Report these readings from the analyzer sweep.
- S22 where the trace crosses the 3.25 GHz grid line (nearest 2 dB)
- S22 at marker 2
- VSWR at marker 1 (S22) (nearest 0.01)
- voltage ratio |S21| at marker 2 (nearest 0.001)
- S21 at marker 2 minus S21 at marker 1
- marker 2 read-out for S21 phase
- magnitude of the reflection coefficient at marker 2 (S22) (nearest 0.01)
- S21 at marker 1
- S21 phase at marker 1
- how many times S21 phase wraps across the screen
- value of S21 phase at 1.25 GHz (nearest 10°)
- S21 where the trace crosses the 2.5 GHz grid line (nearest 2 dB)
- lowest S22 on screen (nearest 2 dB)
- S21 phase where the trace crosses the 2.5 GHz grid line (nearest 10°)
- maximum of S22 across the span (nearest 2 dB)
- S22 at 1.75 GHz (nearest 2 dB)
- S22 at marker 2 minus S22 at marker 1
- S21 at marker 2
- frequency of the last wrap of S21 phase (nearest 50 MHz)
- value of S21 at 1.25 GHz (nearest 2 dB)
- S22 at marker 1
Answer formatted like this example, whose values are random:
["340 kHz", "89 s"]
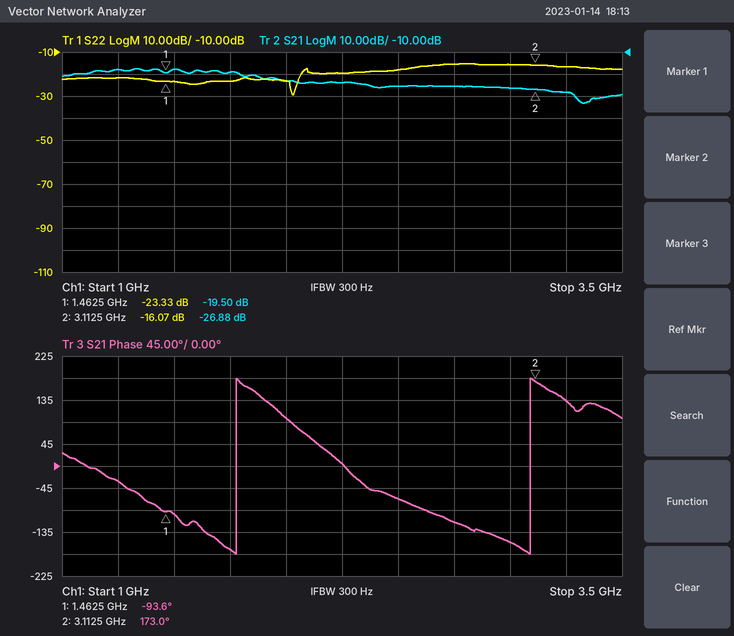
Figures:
["-16 dB", "-16.07 dB", "1.15", "0.045", "-7.38 dB", "173.0°", "0.16", "-19.50 dB", "-93.6°", "2", "-30°", "-26 dB", "-30 dB", "-70°", "-16 dB", "-24 dB", "7.26 dB", "-26.88 dB", "3.10 GHz", "-18 dB", "-23.33 dB"]
